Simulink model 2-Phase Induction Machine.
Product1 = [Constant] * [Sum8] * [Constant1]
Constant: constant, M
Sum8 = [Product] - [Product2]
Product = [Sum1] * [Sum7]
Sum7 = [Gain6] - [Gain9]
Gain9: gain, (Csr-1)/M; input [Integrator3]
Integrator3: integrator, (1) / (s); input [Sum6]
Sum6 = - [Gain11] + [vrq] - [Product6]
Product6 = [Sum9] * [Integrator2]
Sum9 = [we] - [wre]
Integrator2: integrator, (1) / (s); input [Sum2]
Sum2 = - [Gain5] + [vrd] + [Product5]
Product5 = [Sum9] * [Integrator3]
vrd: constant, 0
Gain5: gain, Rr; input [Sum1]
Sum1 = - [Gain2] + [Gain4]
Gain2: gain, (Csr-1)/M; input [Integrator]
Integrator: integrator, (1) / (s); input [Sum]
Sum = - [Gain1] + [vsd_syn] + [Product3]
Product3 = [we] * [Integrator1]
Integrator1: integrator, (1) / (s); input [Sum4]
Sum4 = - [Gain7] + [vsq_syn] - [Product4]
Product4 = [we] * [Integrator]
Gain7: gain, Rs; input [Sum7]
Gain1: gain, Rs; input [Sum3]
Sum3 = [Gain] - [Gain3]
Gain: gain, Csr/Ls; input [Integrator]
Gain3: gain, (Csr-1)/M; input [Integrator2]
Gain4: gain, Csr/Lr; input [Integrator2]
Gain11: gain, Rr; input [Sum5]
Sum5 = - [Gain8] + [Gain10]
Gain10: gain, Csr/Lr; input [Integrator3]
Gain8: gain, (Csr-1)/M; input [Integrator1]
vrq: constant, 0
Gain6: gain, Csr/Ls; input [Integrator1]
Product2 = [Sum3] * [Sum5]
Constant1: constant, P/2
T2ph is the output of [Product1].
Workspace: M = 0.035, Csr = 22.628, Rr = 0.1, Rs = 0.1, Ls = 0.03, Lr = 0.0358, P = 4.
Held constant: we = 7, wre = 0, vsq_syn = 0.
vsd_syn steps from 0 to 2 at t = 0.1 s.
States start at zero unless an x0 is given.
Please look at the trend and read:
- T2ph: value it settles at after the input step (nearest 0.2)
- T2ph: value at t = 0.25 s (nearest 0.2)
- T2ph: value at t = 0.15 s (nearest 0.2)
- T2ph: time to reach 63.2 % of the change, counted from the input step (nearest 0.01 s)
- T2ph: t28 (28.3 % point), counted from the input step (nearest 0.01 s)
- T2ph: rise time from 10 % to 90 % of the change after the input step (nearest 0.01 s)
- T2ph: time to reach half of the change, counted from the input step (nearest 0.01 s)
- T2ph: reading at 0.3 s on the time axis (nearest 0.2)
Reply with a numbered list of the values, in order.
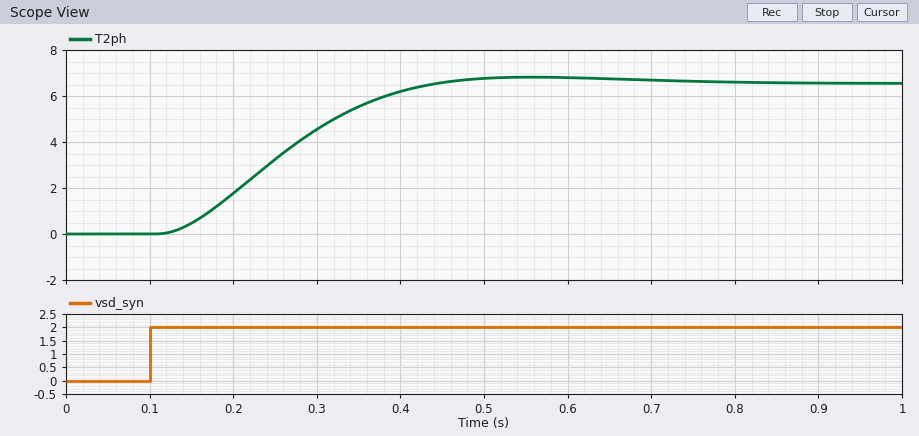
1. 6.6
2. 3.2
3. 0.4
4. 0.18 s
5. 0.10 s
6. 0.22 s
7. 0.15 s
8. 4.6
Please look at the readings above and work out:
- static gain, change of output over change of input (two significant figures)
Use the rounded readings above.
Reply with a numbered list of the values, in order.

1. 3.3
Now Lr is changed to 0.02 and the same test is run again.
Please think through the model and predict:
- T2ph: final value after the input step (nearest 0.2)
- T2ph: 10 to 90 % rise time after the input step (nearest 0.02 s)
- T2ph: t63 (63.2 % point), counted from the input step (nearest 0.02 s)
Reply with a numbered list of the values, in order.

1. 2.4
2. 0.10 s
3. 0.08 s
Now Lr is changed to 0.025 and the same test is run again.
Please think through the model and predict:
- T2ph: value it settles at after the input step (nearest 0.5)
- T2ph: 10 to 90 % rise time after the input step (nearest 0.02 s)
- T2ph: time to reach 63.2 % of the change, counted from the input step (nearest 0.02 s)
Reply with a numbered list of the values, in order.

1. 3.5
2. 0.14 s
3. 0.10 s
